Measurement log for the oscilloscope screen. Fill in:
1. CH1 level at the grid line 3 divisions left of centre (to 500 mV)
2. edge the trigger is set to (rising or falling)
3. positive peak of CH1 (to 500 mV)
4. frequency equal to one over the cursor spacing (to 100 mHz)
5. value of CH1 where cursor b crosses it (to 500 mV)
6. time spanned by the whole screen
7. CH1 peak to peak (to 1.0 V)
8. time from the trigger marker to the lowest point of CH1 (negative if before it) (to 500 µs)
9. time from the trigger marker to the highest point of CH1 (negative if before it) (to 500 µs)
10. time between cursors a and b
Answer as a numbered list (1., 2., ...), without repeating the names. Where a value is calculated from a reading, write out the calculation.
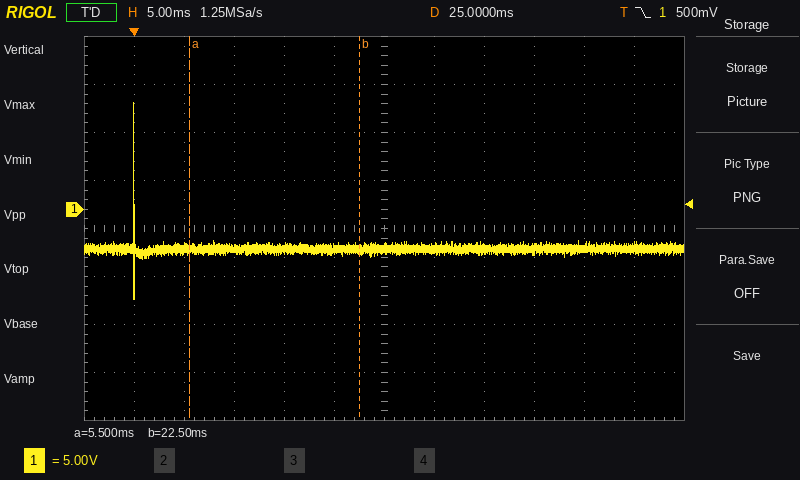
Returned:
1. -4.0 V
2. falling
3. 11.0 V
4. 1 / 17.0 ms ≈ 58.8 Hz
5. -4.0 V
6. 60 ms
7. 20.0 V
8. 0.0 ms
9. 0.0 ms
10. 22.5 ms − (5.5 ms) = 17.0 ms
